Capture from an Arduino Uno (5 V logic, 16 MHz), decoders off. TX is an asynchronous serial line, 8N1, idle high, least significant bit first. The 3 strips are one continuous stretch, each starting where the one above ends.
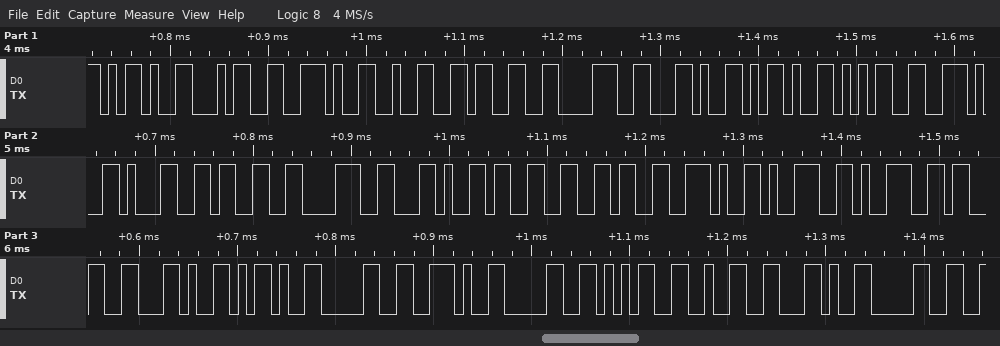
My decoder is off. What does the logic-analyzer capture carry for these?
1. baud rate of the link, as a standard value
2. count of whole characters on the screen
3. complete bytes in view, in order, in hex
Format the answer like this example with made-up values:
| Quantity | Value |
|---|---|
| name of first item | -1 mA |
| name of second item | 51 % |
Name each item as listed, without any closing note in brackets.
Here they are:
| Quantity | Value |
|---|---|
| baud rate of the link, as a standard value | 115200 baud |
| count of whole characters on the screen | 29 |
| complete bytes in view, in order, in hex | 0x2D 0x34 0x2E 0x32 0x33 0x38 0x2C 0x2D 0x35 0x2E 0x31 0x33 0x38 0x2C 0x33 0x36 0x2E 0x39 0x39 0x33 0x2C 0x2D 0x30 0x2E 0x30 0x35 0x32 0x2C 0x30 |
